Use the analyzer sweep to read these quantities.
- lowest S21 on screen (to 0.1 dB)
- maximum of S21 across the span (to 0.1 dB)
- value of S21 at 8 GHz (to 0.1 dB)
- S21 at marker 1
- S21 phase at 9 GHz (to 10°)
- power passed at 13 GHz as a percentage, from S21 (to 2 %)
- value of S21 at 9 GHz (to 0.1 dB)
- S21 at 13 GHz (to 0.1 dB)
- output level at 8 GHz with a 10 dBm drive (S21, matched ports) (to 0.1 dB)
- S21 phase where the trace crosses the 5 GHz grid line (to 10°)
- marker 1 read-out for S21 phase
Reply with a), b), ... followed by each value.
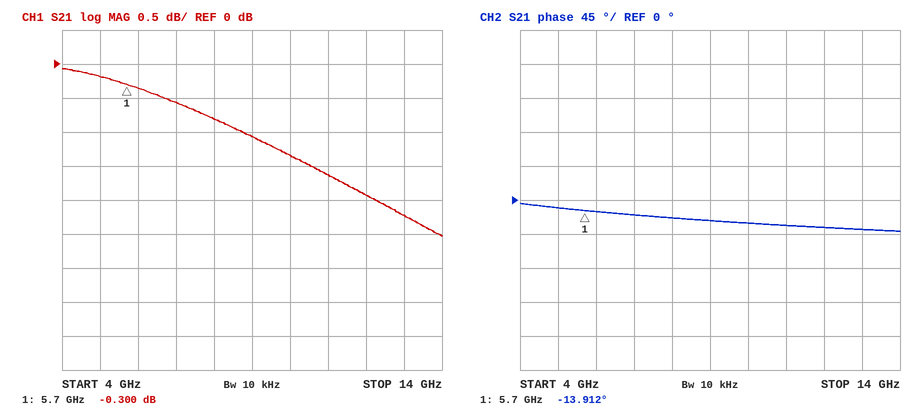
a) -2.5 dB
b) -0.1 dB
c) -0.8 dB
d) -0.300 dB
e) -30°
f) 60 %
g) -1.1 dB
h) -2.2 dB
i) 9.2 dBm
j) -10°
k) -13.912°
